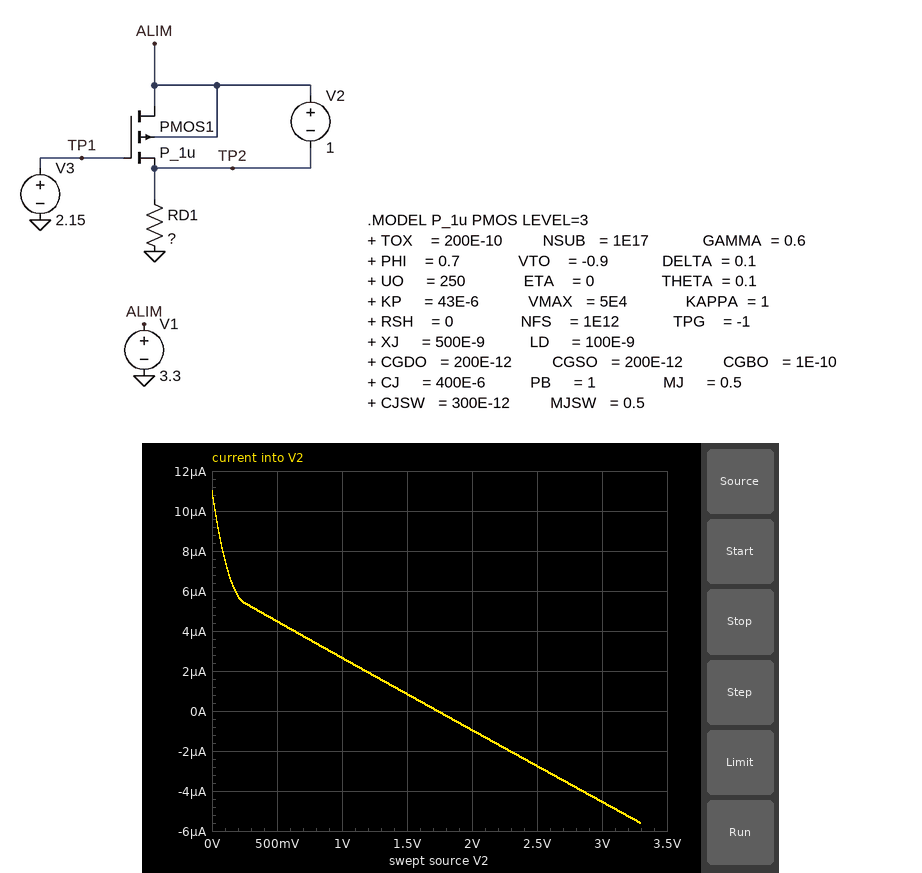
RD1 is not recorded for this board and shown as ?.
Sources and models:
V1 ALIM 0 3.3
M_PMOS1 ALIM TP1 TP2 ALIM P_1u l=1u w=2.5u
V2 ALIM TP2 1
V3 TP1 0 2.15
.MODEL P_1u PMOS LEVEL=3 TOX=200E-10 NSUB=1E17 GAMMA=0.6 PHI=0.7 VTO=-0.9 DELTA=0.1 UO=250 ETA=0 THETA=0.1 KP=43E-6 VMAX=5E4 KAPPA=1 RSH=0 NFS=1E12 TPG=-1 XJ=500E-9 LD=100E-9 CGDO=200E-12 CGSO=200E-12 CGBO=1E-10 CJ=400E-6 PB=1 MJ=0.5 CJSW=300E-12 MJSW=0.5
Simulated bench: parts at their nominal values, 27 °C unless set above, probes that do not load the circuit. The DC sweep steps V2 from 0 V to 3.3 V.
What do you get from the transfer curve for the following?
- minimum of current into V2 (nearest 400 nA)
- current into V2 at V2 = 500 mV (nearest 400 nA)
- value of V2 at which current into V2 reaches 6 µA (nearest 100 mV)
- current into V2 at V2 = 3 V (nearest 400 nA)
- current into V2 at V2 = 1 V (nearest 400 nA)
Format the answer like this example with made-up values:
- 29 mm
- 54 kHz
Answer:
- -5.6 µA
- 4.4 µA
- 200 mV
- -4.4 µA
- 2.8 µA
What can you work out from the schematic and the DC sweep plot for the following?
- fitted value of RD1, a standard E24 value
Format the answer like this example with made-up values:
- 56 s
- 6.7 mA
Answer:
- 300 kΩ
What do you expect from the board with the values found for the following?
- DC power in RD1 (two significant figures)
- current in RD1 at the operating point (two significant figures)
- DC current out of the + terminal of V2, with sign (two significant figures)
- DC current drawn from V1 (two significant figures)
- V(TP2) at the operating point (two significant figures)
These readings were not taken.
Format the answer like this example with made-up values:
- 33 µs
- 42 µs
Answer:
- 18 µW
- 7.7 µA
- -2.7 µA
- 7.7 µA
- 2.3 V
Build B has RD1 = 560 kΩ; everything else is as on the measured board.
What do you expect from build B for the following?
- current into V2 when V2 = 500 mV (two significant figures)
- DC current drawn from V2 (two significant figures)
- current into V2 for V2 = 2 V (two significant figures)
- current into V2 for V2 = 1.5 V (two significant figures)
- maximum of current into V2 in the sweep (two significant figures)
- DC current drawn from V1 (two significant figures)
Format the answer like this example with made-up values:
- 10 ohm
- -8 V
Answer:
- 150 nA
- 900 nA
- -3.0 µA
- -1.9 µA
- 5.9 µA
- 4.1 µA
